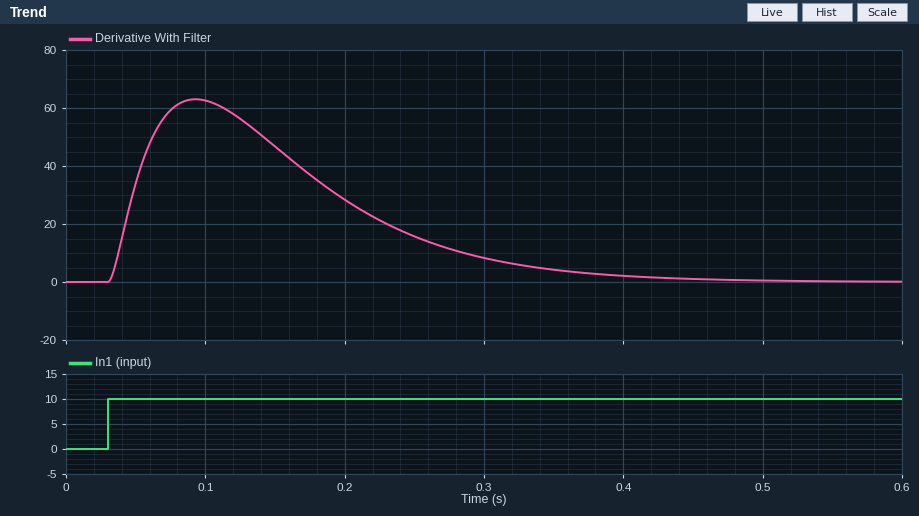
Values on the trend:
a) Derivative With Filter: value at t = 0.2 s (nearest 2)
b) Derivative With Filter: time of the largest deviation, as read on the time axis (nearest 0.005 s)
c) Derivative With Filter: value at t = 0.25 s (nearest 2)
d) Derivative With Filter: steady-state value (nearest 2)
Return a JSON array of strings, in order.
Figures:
["28", "0.095 s", "16", "0"]
